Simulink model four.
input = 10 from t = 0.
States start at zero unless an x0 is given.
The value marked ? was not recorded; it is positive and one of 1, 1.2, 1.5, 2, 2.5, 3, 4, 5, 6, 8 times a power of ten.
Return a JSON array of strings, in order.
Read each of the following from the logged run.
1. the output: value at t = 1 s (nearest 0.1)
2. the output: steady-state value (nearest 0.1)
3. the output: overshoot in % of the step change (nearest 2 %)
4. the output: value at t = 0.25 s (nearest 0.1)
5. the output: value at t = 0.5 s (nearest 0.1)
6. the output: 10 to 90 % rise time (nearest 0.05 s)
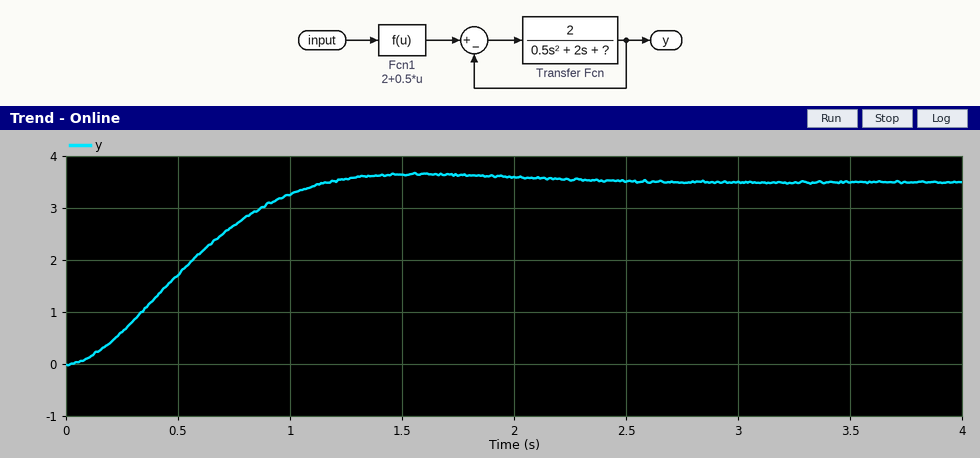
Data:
["3.3", "3.5", "4 %", "0.6", "1.7", "0.75 s"]
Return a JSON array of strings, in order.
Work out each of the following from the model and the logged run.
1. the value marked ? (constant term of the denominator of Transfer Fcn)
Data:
["2"]
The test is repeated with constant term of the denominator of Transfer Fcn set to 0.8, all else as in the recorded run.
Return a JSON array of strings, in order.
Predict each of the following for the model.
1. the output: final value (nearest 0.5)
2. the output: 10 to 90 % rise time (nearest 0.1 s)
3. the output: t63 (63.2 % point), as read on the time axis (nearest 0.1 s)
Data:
["5.0", "1.1 s", "0.8 s"]
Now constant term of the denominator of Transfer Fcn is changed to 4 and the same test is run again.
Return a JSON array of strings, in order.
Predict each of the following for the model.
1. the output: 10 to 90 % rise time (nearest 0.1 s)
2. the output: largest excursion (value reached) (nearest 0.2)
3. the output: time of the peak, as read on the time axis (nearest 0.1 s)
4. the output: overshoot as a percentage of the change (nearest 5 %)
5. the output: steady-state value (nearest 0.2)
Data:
["0.5 s", "2.6", "1.1 s", "10 %", "2.4"]
